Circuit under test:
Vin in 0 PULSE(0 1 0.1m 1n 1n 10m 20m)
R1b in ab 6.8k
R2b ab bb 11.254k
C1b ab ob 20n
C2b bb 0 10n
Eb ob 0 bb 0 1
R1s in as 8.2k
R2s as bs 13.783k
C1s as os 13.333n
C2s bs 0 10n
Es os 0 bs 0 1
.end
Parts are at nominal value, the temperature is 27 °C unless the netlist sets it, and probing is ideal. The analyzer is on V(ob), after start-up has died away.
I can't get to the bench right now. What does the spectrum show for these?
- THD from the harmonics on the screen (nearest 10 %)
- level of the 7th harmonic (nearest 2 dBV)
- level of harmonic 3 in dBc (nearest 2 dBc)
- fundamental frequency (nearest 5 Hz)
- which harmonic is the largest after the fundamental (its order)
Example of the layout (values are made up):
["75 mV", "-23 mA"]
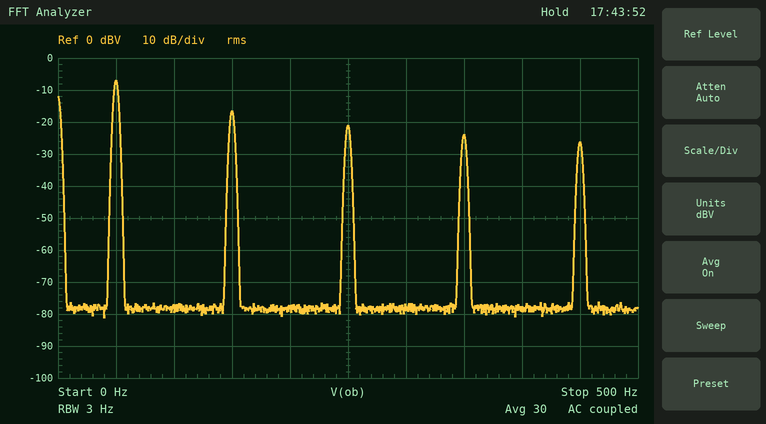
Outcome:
["40 %", "-24 dBV", "-10 dBc", "50 Hz", "3"]
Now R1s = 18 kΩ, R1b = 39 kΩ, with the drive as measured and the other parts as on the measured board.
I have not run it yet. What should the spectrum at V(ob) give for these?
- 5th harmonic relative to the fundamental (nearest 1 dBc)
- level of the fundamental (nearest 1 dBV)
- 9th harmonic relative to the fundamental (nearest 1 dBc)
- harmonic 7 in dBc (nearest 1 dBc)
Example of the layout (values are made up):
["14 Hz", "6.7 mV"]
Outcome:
["-15 dBc", "-7 dBV", "-22 dBc", "-19 dBc"]
